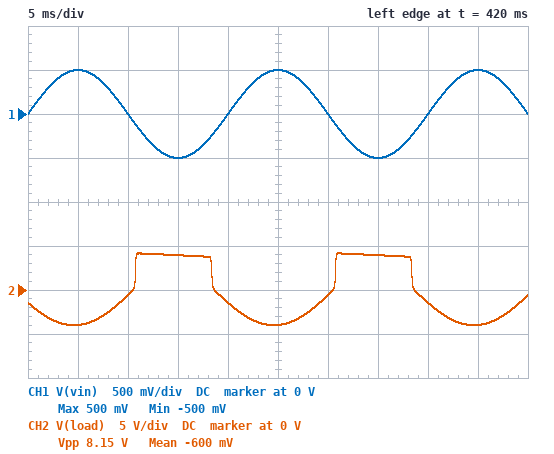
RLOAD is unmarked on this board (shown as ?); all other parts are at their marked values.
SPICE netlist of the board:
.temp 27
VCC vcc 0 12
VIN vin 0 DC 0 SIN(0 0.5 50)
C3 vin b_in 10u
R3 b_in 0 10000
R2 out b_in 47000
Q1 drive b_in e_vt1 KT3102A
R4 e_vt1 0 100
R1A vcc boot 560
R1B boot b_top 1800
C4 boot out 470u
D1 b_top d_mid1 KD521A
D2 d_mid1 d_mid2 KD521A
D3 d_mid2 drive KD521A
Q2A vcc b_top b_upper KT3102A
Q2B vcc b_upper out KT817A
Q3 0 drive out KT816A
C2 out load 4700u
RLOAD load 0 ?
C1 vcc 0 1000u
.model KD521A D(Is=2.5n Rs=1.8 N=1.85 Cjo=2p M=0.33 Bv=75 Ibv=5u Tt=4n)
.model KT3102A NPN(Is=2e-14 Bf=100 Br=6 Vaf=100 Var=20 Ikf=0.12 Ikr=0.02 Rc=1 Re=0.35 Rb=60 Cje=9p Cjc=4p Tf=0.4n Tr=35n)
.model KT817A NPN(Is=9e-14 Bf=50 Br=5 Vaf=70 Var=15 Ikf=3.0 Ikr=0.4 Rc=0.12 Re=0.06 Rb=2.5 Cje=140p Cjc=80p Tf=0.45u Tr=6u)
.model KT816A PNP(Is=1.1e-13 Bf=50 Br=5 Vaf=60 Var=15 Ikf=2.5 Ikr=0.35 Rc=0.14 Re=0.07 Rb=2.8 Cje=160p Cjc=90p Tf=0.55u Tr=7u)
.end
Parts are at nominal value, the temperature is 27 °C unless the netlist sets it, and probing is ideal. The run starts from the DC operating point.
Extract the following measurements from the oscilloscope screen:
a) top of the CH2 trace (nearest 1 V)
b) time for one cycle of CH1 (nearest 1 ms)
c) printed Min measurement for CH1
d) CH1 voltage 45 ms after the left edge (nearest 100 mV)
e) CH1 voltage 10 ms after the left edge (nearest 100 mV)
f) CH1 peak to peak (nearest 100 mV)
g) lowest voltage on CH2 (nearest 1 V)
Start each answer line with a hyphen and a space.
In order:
- 4 V
- 20 ms
- -500 mV
- 500 mV
- 0 V
- 1.0 V
- -4 V
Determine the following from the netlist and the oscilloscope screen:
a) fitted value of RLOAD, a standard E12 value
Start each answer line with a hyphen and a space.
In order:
- 15 Ω
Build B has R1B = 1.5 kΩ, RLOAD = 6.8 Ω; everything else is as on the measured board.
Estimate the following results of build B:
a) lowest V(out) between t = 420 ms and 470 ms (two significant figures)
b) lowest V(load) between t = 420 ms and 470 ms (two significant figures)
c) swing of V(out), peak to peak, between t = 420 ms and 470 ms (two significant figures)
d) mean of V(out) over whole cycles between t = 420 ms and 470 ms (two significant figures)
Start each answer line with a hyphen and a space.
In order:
- 5.8 V
- -2.2 V
- 5.4 V
- 8.0 V
